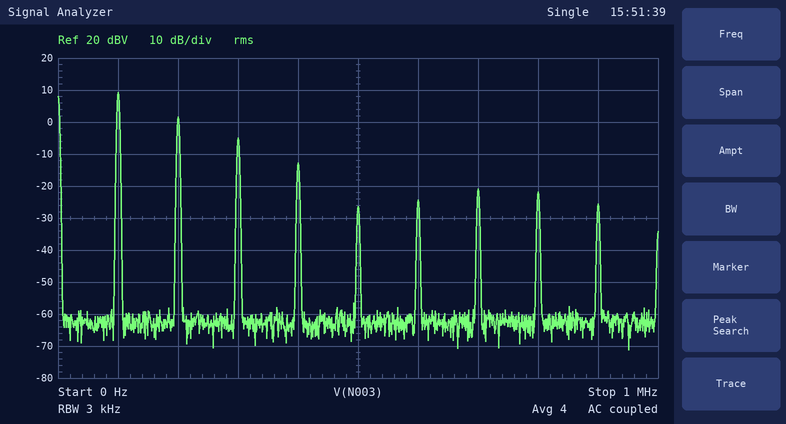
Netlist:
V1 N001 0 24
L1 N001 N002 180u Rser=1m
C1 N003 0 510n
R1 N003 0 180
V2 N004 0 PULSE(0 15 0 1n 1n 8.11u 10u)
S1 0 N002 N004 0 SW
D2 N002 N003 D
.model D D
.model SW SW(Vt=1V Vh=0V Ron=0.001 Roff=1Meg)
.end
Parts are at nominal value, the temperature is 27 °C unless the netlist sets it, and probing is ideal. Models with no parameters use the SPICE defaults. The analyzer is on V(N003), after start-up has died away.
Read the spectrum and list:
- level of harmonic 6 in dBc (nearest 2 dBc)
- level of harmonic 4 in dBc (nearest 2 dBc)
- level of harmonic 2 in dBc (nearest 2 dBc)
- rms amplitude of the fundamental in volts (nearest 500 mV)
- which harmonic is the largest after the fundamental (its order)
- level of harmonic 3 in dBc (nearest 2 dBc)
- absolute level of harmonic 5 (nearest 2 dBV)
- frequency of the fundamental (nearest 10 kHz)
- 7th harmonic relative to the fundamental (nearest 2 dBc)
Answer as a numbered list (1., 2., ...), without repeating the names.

1. -34 dBc
2. -22 dBc
3. -8 dBc
4. 3.0 V
5. 2
6. -14 dBc
7. -26 dBV
8. 100 kHz
9. -30 dBc
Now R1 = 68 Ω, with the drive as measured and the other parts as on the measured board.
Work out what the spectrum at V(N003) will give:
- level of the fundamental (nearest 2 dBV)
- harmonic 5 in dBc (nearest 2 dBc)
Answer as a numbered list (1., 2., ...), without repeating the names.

1. 18 dBV
2. -38 dBc
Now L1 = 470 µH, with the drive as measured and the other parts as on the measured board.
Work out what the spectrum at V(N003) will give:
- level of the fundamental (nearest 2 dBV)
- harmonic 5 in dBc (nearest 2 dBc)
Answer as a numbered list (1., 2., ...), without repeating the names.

1. 10 dBV
2. -38 dBc
